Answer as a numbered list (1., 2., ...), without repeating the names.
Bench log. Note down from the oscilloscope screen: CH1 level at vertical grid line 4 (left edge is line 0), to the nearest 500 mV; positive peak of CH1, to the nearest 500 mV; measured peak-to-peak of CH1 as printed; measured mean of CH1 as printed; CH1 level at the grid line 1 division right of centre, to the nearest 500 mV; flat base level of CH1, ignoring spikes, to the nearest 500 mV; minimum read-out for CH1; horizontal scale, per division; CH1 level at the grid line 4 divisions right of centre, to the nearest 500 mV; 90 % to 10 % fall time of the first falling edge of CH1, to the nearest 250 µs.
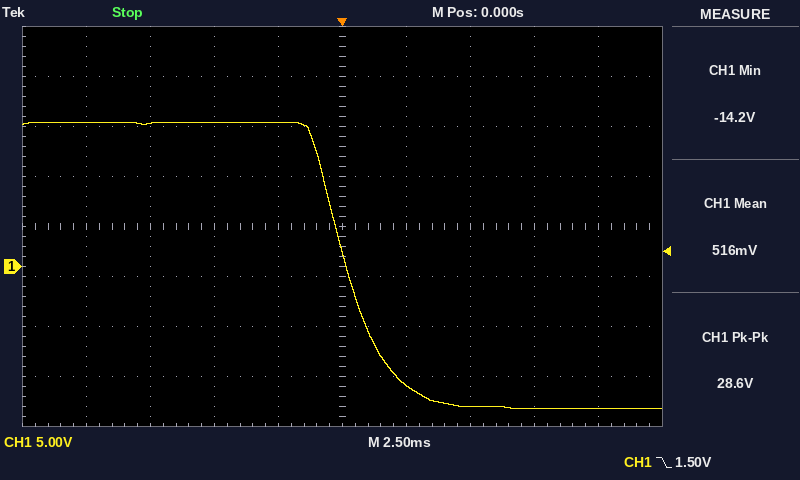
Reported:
1. 14.5 V
2. 14.5 V
3. 28.6 V
4. 516 mV
5. -12.0 V
6. -14.0 V
7. -14.2 V
8. 2.5 ms
9. -14.0 V
10. 3.25 ms
